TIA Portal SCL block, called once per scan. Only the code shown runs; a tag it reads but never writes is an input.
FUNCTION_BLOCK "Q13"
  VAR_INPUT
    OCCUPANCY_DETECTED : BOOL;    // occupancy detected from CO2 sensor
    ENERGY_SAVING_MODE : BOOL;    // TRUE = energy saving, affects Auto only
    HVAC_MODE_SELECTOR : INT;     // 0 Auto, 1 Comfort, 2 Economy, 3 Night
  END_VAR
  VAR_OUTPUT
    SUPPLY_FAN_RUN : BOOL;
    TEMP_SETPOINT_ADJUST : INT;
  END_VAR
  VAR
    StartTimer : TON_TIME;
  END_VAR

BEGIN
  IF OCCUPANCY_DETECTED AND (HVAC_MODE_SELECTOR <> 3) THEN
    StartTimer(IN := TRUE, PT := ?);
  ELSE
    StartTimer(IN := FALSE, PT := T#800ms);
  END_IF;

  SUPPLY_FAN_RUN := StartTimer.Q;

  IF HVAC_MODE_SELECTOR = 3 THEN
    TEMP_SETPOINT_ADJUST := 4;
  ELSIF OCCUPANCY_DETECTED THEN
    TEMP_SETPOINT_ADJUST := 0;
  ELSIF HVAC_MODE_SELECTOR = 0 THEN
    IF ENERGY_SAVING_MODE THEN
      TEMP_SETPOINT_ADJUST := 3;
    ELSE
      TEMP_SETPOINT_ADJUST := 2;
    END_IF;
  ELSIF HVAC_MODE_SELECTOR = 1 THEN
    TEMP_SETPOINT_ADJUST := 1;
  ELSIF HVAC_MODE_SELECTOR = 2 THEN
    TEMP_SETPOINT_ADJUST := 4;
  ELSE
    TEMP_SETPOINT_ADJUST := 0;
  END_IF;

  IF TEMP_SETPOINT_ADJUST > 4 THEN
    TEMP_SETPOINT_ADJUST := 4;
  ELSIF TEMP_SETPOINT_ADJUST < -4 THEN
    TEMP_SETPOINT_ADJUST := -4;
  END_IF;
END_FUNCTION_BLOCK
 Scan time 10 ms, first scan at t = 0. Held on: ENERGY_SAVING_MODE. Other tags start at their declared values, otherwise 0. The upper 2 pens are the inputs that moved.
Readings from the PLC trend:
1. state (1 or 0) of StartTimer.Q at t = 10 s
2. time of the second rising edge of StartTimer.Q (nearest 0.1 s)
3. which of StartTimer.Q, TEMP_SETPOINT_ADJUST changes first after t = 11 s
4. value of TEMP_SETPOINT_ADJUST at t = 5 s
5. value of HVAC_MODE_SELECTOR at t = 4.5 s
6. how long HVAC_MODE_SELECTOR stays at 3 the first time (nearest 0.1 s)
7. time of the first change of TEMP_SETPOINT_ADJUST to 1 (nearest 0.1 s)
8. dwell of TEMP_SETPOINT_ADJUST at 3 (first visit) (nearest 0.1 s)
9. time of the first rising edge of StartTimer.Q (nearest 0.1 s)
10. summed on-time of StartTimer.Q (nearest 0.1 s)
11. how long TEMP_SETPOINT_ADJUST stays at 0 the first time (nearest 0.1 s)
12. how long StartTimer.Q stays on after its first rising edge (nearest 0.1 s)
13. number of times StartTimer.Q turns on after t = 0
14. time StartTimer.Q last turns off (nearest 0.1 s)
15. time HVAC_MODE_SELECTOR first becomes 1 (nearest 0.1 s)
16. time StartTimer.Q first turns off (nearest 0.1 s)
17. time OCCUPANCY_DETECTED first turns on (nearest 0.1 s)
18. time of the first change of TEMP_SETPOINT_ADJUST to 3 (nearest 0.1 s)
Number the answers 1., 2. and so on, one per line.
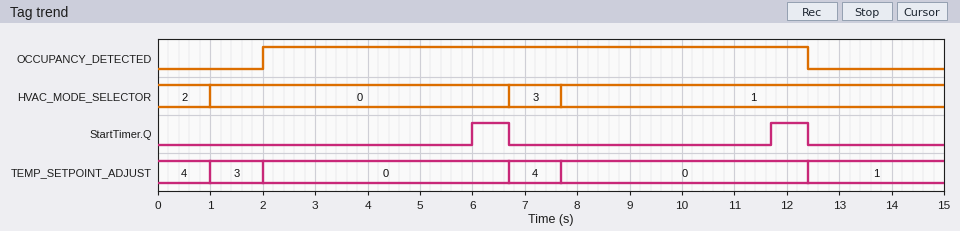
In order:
1. 0
2. 11.7 s
3. StartTimer.Q
4. 0
5. 0
6. 1.0 s
7. 12.4 s
8. 1.0 s
9. 6.0 s
10. 1.4 s
11. 4.7 s
12. 0.7 s
13. 2
14. 12.4 s
15. 7.7 s
16. 6.7 s
17. 2.0 s
18. 1.0 s
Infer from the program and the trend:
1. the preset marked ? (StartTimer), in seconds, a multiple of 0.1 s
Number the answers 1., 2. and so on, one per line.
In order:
1. 4.0 s
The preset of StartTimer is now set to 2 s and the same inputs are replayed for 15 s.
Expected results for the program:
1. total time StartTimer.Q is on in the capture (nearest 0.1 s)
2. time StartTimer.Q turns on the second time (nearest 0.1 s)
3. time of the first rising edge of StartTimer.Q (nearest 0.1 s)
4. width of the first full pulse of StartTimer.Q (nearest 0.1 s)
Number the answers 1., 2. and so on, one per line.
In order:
1. 5.4 s
2. 9.7 s
3. 4.0 s
4. 2.7 s
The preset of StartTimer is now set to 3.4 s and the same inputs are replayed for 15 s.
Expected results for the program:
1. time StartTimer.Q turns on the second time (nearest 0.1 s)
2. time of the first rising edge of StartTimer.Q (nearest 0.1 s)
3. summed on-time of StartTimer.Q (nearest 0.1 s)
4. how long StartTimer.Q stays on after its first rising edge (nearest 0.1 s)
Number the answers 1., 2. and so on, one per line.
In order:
1. 11.1 s
2. 5.4 s
3. 2.6 s
4. 1.3 s
